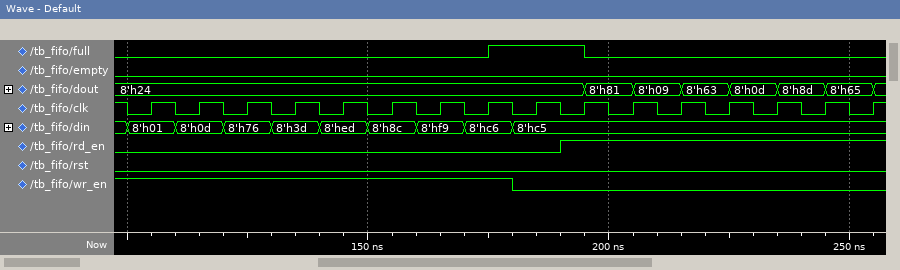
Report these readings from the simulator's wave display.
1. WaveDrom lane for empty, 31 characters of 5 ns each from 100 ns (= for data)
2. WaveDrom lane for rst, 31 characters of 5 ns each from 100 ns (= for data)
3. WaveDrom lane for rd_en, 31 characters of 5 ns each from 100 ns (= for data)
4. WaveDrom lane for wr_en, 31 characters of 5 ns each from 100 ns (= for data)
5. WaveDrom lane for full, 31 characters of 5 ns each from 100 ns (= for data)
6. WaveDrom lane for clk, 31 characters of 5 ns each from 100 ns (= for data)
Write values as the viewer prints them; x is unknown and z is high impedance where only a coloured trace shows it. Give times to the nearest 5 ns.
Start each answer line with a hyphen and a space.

- {name: 'empty', wave: '0..............................'}
- {name: 'rst', wave: '0..............................'}
- {name: 'rd_en', wave: '0.................1............'}
- {name: 'wr_en', wave: '1...............0..............'}
- {name: 'full', wave: '0..............1...0...........'}
- {name: 'clk', wave: '0101010101010101010101010101010'}
